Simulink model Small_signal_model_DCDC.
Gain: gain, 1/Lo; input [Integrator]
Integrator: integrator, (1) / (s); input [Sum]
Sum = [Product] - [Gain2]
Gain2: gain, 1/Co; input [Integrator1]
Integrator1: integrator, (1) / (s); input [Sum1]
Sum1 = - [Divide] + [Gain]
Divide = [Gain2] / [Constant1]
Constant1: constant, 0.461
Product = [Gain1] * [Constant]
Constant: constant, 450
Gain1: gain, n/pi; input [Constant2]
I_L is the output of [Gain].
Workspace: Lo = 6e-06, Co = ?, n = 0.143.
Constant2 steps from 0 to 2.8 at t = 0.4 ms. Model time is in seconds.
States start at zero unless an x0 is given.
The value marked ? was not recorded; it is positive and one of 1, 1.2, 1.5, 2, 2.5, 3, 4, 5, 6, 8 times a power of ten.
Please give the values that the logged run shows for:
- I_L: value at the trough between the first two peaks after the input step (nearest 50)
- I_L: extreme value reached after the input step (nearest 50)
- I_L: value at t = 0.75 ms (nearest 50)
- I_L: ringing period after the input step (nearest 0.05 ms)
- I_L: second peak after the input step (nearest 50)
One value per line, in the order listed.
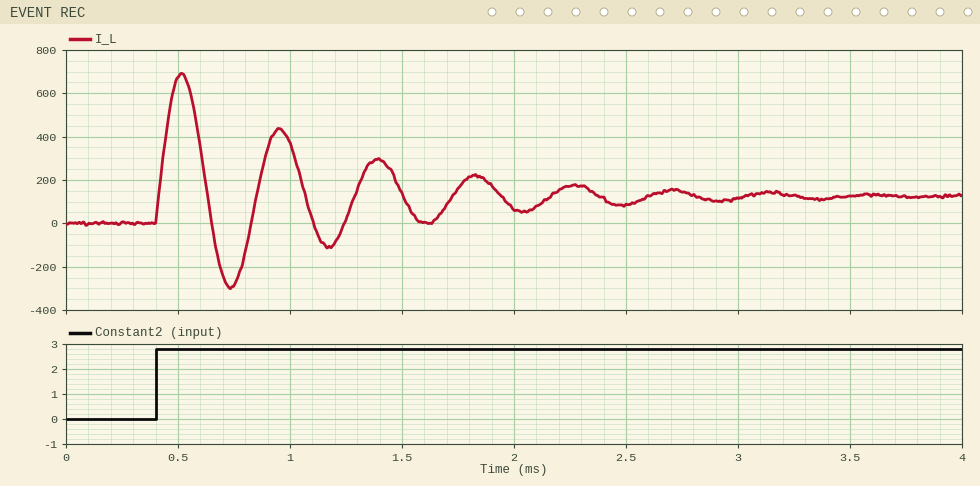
-300
700
-300
0.45 ms
450
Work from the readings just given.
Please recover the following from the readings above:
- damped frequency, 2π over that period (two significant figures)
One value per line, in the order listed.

14 rad/ms
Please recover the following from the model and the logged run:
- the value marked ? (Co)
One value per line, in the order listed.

0.0008
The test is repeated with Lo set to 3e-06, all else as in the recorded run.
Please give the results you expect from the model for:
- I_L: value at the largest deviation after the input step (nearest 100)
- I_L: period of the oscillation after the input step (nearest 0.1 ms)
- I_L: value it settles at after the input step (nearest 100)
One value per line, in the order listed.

1000
0.3 ms
100
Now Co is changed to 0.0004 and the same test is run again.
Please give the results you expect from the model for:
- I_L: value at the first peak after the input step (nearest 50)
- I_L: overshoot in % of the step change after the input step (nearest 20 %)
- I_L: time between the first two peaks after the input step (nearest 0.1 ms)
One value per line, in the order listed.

500
300 %
0.3 ms
